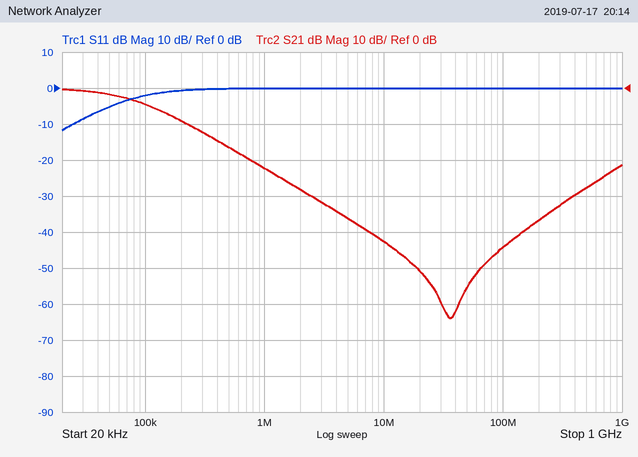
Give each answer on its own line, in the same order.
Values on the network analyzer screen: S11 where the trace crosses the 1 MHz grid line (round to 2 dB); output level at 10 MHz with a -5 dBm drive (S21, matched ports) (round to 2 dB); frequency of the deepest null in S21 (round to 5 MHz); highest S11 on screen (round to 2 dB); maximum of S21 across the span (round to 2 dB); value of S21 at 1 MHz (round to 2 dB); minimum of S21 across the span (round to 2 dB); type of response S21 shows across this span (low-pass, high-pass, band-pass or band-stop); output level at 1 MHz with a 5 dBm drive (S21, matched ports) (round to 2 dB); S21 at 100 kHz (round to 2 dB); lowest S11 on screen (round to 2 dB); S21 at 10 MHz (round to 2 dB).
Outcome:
0 dB
-48 dBm
35 MHz
0 dB
0 dB
-22 dB
-64 dB
low-pass
-18 dBm
-4 dB
-12 dB
-42 dB
